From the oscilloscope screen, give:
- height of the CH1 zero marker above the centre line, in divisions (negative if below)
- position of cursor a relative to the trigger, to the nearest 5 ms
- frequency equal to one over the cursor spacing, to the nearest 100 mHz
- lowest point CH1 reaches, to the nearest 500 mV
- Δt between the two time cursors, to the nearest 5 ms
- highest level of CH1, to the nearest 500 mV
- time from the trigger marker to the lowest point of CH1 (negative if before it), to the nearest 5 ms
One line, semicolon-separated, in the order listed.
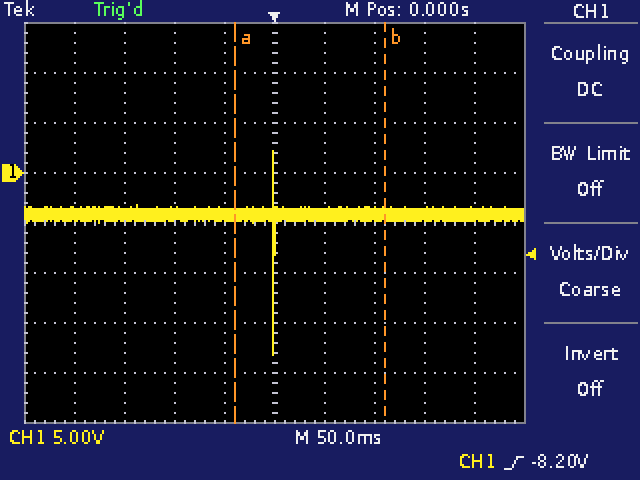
+1.0 div; -40 ms; 6.7 Hz; -18.0 V; 150 ms; 2.0 V; 0 ms
